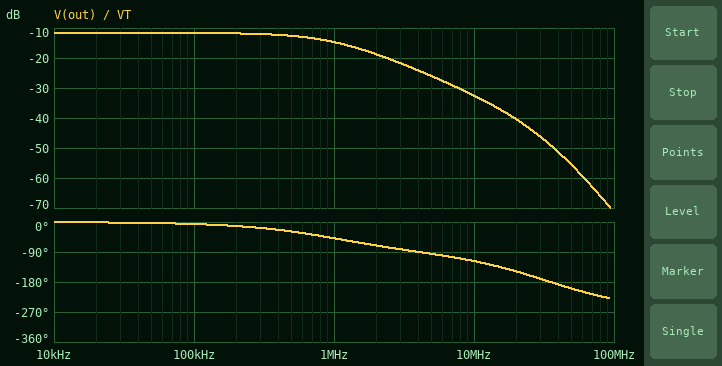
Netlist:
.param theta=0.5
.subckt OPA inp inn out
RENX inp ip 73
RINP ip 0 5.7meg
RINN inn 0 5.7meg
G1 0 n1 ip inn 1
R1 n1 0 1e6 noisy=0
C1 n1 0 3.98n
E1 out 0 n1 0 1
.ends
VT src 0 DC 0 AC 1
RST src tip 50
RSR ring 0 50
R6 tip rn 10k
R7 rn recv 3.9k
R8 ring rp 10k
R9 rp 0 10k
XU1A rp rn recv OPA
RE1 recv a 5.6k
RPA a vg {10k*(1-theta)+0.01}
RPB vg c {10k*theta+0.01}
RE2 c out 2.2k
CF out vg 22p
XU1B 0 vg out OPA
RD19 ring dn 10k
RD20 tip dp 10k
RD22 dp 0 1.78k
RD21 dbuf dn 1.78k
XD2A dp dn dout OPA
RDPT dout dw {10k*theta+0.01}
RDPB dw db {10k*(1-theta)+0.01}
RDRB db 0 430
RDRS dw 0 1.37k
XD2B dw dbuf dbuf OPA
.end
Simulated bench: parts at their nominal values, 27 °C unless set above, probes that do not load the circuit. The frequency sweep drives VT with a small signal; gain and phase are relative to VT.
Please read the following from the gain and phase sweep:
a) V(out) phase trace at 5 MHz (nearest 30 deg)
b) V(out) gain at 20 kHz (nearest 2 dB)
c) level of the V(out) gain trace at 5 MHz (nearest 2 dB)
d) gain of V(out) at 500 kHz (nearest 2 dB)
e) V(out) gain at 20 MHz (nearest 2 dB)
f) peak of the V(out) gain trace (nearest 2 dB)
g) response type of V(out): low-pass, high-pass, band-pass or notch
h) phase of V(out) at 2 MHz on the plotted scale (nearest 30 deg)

-90 deg
-12 dB
-26 dB
-12 dB
-40 dB
-12 dB
low-pass
-60 deg
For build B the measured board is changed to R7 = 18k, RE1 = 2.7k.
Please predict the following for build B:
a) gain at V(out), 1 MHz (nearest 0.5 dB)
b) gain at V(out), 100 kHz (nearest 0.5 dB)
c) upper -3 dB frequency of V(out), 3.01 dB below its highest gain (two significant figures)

1.5 dB
4.5 dB
980 kHz
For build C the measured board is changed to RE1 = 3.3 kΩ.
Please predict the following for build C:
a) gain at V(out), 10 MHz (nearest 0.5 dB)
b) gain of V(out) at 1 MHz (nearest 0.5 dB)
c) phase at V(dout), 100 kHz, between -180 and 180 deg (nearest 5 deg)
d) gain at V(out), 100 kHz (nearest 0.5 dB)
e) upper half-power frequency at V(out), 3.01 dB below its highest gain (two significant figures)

-30.5 dB
-12.5 dB
0 deg
-9.5 dB
980 kHz
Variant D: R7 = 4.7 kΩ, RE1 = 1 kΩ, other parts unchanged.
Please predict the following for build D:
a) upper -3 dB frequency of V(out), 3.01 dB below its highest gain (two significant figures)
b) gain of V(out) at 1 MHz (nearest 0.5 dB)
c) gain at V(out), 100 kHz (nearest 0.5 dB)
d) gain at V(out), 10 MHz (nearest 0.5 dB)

970 kHz
-8.0 dB
-5.0 dB
-26.0 dB
